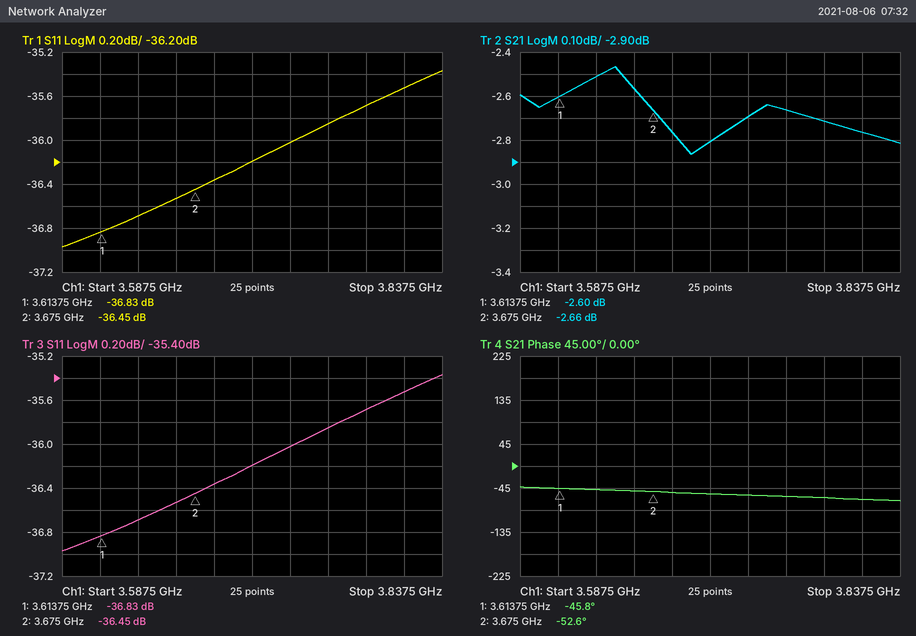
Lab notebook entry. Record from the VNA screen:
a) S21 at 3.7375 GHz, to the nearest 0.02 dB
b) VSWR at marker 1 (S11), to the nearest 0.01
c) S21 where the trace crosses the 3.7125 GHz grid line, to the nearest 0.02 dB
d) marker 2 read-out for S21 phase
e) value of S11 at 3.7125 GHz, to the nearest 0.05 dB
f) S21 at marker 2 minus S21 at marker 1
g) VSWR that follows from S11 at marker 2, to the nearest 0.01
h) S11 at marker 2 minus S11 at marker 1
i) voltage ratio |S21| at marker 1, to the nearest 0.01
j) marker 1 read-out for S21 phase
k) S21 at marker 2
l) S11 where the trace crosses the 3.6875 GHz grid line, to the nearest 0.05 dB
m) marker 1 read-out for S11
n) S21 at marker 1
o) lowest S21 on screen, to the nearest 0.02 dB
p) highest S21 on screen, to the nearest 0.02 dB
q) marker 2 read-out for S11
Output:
-2.70 dB
1.03
-2.80 dB
-52.6°
-36.20 dB
-0.06 dB
1.03
0.38 dB
0.74
-45.8°
-2.66 dB
-36.35 dB
-36.83 dB
-2.60 dB
-2.86 dB
-2.46 dB
-36.45 dB
